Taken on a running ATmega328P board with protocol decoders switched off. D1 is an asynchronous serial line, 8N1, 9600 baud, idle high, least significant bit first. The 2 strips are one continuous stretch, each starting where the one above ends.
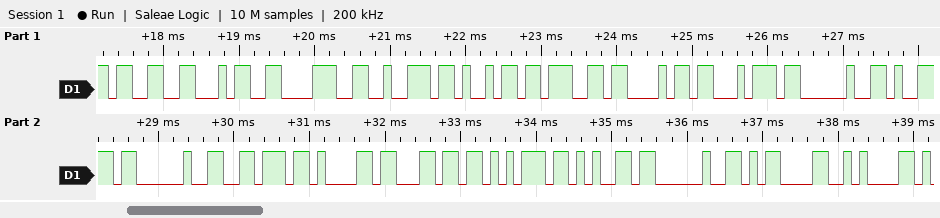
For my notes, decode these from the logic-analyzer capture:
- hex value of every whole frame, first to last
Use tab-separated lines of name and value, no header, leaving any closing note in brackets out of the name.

hex value of every whole frame, first to last	0x33 0x34 0x38 0x72 0x69 0x67 0x68 0x74 0x20 0x79 0x20 0x76 0x61 0x6C 0x75 0x65 0x20 0x0D 0x0A
